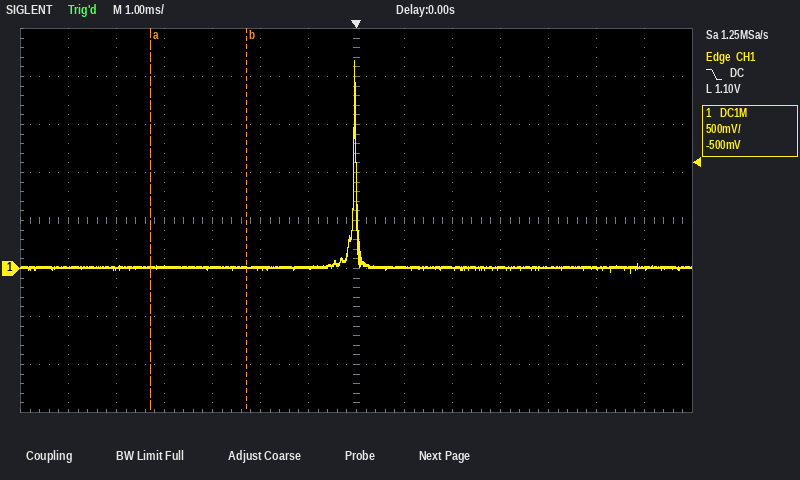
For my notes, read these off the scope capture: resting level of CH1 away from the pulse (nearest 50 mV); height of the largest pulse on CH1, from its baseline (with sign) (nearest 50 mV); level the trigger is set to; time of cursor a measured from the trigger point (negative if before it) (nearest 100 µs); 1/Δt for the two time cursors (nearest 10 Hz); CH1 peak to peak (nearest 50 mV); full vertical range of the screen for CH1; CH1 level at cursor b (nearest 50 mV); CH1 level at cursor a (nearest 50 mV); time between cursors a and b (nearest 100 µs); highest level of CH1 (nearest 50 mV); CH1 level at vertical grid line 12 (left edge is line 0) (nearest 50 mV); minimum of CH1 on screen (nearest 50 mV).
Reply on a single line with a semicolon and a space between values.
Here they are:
0 mV; +2.15 V; 1.10 V; -4.3 ms; 500 Hz; 2.20 V; 4 V; 0 mV; 0 mV; 2.0 ms; 2.15 V; 0 mV; -50 mV
